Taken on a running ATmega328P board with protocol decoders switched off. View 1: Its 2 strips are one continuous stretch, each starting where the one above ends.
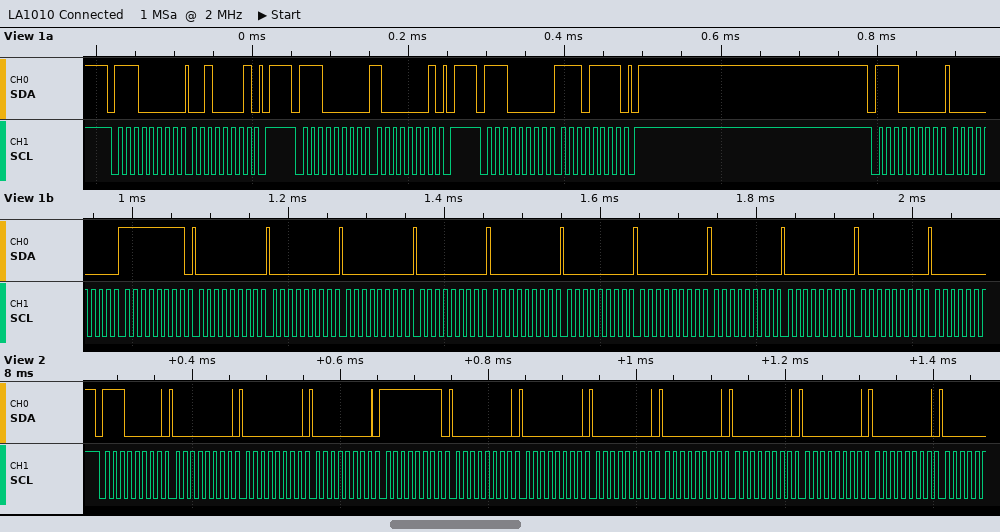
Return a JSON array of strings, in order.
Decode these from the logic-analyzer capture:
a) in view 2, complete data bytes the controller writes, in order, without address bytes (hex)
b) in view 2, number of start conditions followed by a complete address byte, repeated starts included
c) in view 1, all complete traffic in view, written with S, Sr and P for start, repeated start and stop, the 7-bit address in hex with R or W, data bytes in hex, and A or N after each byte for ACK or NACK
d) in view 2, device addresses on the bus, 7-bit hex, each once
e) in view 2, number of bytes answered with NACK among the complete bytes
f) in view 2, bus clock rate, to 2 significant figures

["00 00 00 FF 00 00 00 00 00 00 00", "1", "S 70W A 21 A P S 70W A 81 A P S 70W A EF A P S 70W A 00 A FF A 00 A 00 A 00 A 00 A 00 A 00 A 00 A 00 A 00 A 00 A", "0x70", "0", "100 kHz"]
